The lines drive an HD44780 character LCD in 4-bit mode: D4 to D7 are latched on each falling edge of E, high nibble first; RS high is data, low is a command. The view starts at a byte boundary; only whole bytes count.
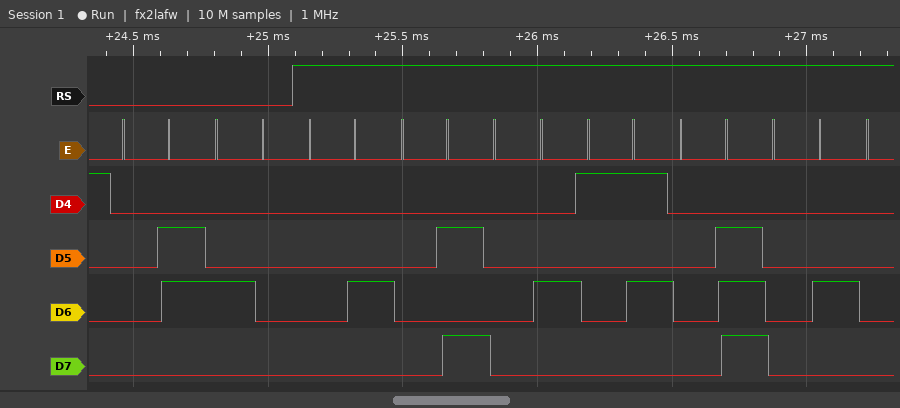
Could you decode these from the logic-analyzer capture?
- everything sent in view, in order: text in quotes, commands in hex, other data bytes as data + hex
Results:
0x06 0x40 data 04 0A 04 15 0E 04
